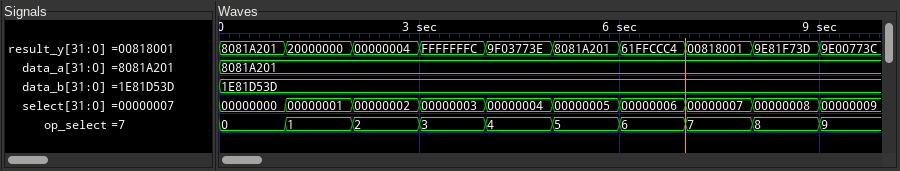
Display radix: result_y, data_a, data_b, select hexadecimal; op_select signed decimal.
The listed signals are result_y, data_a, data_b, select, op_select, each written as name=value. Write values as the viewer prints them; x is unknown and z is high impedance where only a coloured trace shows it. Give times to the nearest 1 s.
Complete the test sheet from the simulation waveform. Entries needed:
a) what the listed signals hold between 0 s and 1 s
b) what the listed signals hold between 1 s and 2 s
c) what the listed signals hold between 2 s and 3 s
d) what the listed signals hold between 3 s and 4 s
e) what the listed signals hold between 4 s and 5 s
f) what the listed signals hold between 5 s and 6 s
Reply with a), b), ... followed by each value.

a) result_y=8081A201, data_a=8081A201, data_b=1E81D53D, select=00000000, op_select=0
b) result_y=20000000, data_a=8081A201, data_b=1E81D53D, select=00000001, op_select=1
c) result_y=00000004, data_a=8081A201, data_b=1E81D53D, select=00000002, op_select=2
d) result_y=FFFFFFFC, data_a=8081A201, data_b=1E81D53D, select=00000003, op_select=3
e) result_y=9F03773E, data_a=8081A201, data_b=1E81D53D, select=00000004, op_select=4
f) result_y=8081A201, data_a=8081A201, data_b=1E81D53D, select=00000005, op_select=5
